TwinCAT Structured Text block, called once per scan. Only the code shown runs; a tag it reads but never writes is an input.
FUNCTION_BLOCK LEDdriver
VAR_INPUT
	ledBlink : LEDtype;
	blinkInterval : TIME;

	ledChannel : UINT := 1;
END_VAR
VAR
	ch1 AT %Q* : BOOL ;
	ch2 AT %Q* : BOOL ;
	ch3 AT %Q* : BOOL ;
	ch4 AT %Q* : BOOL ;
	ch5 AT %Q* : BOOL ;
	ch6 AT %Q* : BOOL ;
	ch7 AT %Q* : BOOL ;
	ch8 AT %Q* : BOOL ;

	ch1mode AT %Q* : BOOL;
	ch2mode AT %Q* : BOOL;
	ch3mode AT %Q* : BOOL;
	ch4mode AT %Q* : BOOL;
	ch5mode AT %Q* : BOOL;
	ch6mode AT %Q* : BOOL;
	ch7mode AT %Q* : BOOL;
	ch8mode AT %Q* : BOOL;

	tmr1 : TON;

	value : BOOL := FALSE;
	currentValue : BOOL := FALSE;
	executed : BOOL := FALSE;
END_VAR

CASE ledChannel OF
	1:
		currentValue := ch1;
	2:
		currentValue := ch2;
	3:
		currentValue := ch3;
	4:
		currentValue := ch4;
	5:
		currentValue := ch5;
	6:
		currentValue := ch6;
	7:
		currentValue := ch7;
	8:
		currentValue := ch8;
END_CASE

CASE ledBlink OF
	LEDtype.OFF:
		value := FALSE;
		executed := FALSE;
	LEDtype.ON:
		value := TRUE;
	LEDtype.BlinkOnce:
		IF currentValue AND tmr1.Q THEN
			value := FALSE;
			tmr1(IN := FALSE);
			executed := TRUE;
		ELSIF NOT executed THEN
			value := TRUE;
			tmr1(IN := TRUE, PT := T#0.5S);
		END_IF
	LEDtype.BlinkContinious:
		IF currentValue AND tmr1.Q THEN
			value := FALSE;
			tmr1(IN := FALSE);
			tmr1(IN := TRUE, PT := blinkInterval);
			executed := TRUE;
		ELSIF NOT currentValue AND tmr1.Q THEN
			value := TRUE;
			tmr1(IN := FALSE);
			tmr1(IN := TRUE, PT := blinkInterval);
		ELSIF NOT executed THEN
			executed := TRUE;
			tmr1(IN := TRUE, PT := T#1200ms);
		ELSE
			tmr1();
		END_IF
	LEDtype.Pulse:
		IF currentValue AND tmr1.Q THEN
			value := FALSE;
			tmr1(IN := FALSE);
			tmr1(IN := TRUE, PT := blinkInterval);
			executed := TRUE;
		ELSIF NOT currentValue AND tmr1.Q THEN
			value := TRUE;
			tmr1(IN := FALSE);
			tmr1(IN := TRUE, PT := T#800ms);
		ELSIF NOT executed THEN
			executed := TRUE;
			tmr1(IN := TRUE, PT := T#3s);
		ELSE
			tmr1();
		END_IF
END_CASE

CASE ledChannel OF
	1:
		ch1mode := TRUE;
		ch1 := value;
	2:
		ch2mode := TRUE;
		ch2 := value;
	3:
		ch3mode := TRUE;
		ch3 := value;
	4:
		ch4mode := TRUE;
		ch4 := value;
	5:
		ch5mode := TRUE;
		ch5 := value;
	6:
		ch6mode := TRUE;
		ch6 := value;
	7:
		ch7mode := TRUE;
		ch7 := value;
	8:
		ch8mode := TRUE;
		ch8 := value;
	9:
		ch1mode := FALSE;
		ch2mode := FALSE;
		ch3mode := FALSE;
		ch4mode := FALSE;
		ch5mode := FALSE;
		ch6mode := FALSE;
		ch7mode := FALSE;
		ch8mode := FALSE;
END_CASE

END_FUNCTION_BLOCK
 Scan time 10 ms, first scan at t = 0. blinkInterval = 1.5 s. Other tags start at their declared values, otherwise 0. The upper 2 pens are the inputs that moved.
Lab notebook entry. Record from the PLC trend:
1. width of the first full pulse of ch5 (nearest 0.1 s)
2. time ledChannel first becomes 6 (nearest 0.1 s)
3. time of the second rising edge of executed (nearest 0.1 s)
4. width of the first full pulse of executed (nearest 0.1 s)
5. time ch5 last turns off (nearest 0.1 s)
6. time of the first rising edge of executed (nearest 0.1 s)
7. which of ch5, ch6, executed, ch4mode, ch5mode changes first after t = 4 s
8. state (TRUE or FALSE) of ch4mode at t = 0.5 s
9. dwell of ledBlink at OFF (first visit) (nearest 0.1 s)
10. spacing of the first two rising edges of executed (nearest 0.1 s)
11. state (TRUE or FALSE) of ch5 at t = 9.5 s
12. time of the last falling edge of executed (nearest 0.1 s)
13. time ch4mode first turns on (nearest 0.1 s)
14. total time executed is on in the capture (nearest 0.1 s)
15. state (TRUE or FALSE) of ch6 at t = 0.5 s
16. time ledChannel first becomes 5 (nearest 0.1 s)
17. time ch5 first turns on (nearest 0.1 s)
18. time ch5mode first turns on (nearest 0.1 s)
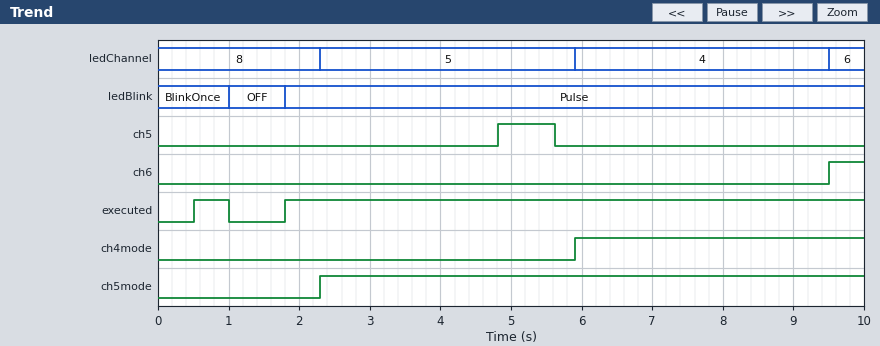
0.8 s
9.5 s
1.8 s
0.5 s
5.6 s
0.5 s
ch5
FALSE
0.8 s
1.3 s
FALSE
1.0 s
5.9 s
8.7 s
FALSE
2.3 s
4.8 s
2.3 s
